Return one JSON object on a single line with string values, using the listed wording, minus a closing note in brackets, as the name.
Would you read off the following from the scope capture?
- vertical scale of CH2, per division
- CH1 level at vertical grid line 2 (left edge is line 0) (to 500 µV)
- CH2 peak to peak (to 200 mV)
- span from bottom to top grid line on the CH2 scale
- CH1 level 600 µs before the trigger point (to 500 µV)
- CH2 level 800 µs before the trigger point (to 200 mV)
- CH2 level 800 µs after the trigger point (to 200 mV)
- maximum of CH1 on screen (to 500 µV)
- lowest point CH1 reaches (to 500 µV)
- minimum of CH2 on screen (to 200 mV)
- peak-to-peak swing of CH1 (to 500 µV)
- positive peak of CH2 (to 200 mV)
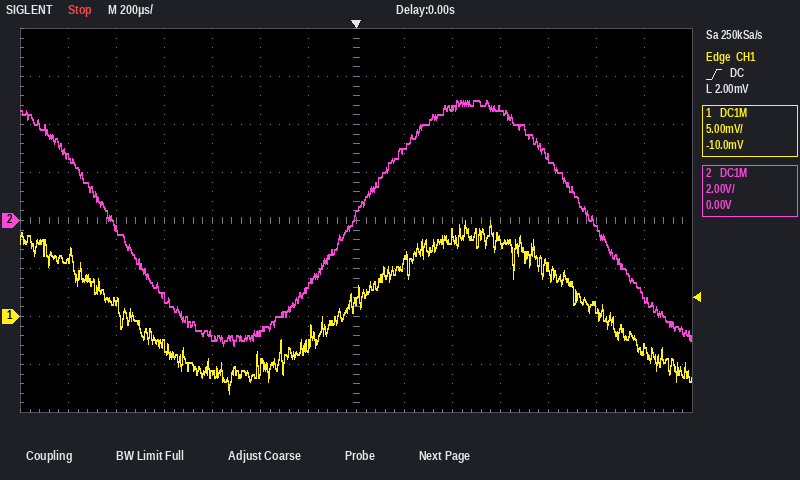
{"vertical scale of CH2, per division": "2 V", "CH1 level at vertical grid line 2 (left edge is line 0)": "1.5 mV", "CH2 peak to peak": "10.2 V", "span from bottom to top grid line on the CH2 scale": "16 V", "CH1 level 600 µs before the trigger point": "-6.0 mV", "CH2 level 800 µs before the trigger point": "-3.2 V", "CH2 level 800 µs after the trigger point": "2.6 V", "maximum of CH1 on screen": "10.0 mV", "lowest point CH1 reaches": "-8.0 mV", "minimum of CH2 on screen": "-5.2 V", "peak-to-peak swing of CH1": "18.0 mV", "positive peak of CH2": "5.0 V"}
